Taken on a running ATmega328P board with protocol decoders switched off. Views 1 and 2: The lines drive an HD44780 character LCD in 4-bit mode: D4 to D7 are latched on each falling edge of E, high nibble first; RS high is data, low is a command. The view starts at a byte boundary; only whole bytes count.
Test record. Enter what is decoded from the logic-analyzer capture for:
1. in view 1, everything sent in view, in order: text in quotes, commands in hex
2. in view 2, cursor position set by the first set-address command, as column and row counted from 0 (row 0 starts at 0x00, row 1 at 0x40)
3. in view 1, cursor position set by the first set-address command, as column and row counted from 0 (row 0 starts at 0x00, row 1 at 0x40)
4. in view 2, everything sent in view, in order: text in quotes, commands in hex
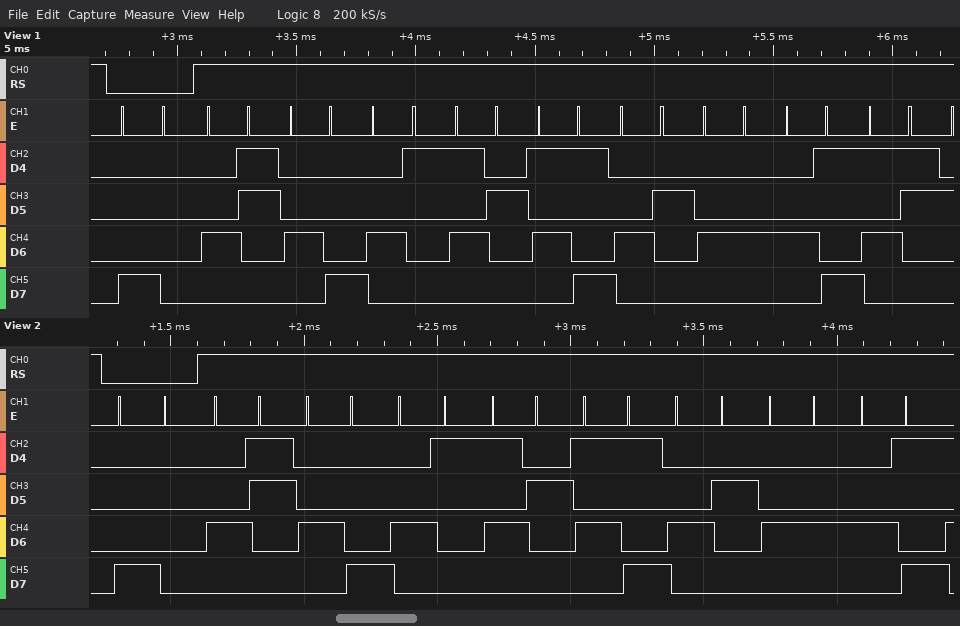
0x80 "CHARYBDIS"
column 0, row 0
column 0, row 0
0x80 "CHARYBDI"
